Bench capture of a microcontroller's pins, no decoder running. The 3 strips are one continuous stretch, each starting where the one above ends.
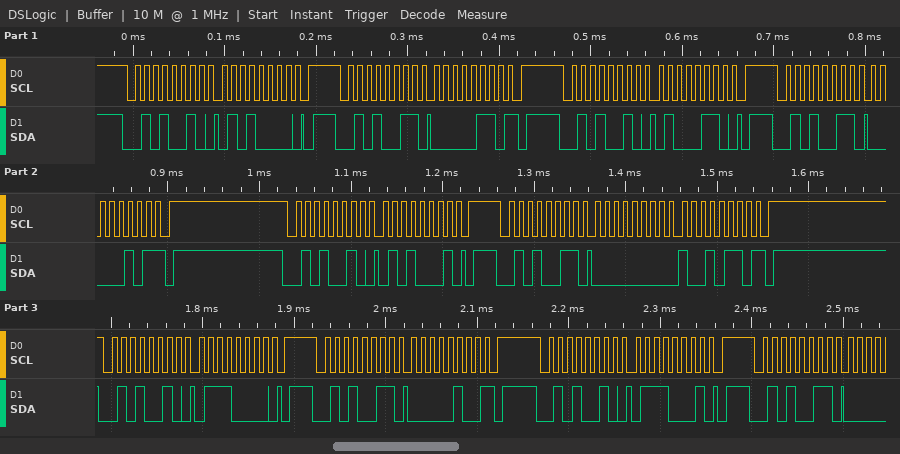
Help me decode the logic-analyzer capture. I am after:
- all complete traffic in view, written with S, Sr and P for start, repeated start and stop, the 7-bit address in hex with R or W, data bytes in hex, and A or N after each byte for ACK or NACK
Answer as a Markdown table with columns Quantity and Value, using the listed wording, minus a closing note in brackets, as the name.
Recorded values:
| Quantity | Value |
|---|---|
| all complete traffic in view, written with S, Sr and P for start, repeated start and stop, the 7-bit address in hex with R or W, data bytes in hex, and A or N after each byte for ACK or NACK | S 29W A 50 A P S 29R A 06 N P S 29W A 46 A P S 29R A 05 N P S 29W A 51 A P S 29R A 00 A 96 N P S 29W A 70 A P S 29R A 04 N P S 29W A 71 A P S 29R A |
